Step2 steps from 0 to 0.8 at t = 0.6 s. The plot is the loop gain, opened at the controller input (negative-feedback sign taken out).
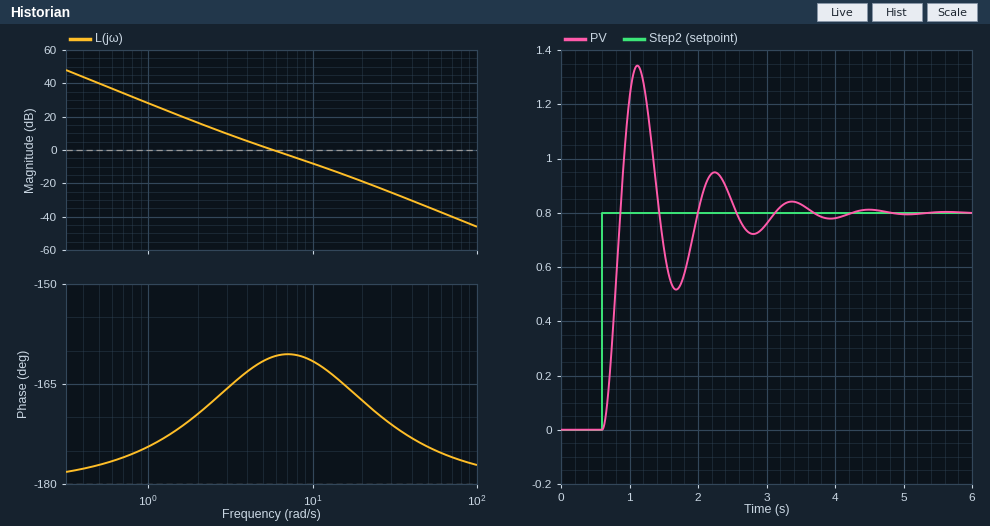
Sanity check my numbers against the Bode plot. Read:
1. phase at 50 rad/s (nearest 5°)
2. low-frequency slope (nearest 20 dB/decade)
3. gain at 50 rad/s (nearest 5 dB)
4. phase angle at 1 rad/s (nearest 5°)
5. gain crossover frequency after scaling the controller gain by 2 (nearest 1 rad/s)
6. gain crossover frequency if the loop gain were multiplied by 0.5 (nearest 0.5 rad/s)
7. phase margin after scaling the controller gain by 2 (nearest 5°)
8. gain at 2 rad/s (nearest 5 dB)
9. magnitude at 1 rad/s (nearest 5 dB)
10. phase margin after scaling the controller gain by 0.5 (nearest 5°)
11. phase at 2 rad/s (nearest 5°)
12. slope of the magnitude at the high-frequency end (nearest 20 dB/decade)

-175°
-40 dB/decade
-35 dB
-175°
9 rad/s
4.0 rad/s
20°
15 dB
30 dB
15°
-170°
-40 dB/decade
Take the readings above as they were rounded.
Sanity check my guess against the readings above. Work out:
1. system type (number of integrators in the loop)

2
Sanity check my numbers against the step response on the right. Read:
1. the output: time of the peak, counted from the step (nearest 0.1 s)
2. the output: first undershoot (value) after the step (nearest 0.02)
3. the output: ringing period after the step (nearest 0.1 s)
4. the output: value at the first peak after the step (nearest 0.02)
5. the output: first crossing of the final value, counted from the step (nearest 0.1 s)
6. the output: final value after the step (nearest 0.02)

0.5 s
0.52
1.1 s
1.34
0.3 s
0.80
